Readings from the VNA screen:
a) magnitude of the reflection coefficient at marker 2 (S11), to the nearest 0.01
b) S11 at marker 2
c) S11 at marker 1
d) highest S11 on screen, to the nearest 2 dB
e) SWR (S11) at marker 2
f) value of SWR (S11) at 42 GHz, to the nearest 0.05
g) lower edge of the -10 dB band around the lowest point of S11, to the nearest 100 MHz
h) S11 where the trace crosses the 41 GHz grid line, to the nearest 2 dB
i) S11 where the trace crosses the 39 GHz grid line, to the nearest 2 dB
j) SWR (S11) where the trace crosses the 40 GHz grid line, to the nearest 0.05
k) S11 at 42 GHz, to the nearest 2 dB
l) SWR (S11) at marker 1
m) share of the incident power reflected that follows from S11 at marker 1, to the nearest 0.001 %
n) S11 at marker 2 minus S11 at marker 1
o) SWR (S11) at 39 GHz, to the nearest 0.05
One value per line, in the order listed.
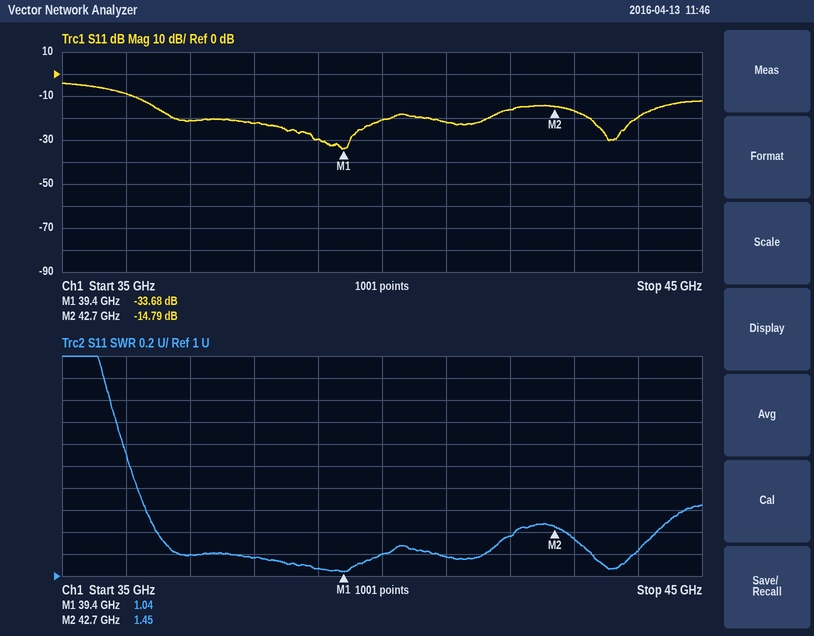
0.18
-14.79 dB
-33.68 dB
-4 dB
1.45
1.35
36.1 GHz
-22 dB
-30 dB
1.20
-16 dB
1.04
0.043 %
18.89 dB
1.05
